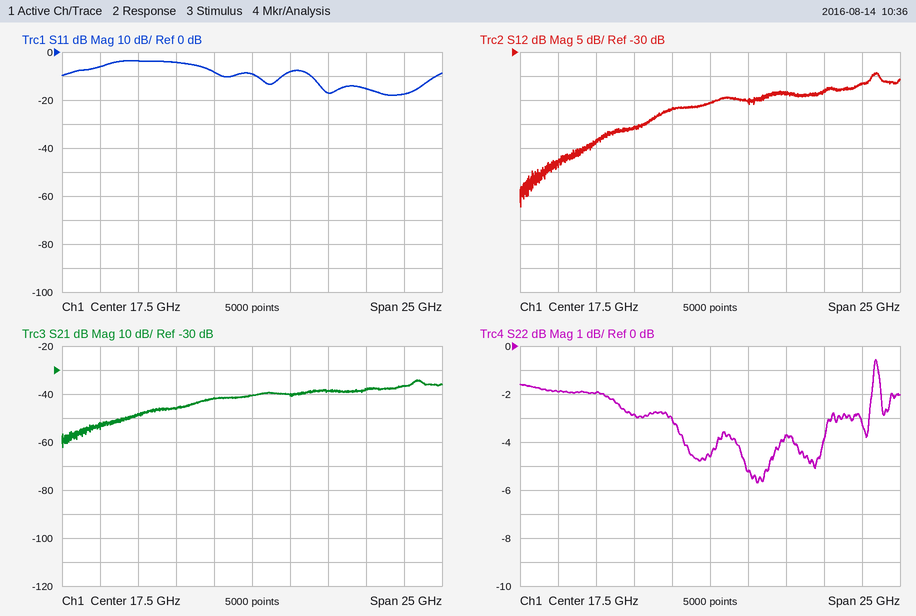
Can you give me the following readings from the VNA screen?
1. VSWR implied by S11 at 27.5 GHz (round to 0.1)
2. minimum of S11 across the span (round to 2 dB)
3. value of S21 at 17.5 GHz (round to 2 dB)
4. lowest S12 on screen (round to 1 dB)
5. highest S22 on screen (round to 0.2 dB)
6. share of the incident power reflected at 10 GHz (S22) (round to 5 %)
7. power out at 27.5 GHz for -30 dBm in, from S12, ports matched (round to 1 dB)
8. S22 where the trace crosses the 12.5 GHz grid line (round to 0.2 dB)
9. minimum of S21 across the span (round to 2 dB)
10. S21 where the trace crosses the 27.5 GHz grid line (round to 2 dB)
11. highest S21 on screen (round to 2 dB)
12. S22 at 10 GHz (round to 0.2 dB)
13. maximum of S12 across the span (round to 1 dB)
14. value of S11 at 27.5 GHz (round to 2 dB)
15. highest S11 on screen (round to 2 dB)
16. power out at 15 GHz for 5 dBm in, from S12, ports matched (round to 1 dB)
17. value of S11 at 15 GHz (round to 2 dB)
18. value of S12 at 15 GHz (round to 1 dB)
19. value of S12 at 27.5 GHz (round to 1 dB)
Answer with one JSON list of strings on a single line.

["1.3", "-18 dB", "-40 dB", "-62 dB", "-0.6 dB", "65 %", "-67 dBm", "-2.8 dB", "-62 dB", "-36 dB", "-34 dB", "-2.0 dB", "-34 dB", "-18 dB", "-4 dB", "-37 dBm", "-8 dB", "-42 dB", "-37 dB"]
